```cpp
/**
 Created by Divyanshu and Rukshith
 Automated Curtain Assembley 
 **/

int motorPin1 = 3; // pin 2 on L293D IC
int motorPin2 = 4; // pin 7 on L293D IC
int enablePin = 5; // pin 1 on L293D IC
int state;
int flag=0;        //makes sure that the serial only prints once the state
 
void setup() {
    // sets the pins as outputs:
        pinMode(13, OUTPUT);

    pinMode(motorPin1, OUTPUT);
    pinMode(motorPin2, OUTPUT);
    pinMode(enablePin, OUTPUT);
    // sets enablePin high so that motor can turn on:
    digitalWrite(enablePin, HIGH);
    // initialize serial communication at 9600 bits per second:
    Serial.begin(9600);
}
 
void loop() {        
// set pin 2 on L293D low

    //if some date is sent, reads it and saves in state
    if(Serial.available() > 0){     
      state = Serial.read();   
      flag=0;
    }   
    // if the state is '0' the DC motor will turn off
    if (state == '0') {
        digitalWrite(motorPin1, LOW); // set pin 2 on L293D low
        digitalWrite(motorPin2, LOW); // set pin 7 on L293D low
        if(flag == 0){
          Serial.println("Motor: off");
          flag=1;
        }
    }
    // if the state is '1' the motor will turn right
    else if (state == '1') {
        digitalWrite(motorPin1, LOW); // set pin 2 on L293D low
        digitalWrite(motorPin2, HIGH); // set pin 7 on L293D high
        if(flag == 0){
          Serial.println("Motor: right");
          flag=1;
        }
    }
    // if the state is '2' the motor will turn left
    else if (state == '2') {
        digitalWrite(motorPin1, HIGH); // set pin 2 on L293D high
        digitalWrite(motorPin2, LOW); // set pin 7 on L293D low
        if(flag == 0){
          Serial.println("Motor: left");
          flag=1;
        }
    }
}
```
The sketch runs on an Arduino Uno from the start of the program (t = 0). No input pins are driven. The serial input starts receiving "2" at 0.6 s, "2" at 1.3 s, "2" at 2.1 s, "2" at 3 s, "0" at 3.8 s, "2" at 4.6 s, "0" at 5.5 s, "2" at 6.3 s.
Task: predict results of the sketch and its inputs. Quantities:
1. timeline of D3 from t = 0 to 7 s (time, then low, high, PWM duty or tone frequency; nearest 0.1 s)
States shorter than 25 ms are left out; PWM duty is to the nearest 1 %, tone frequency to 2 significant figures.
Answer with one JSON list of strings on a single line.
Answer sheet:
["0 s low; 0.6 s high; 3.8 s low; 4.6 s high; 5.5 s low; 6.3 s high"]
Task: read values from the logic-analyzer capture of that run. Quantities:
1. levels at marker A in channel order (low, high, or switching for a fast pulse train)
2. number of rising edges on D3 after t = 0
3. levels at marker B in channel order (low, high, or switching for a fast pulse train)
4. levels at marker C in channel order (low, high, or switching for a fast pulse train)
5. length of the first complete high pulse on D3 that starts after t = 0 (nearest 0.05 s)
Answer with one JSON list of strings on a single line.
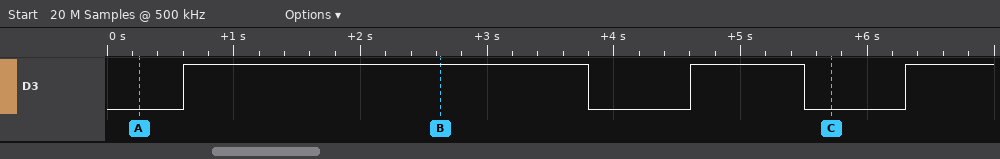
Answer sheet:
["D3 low", "3", "D3 high", "D3 low", "3.20 s"]
